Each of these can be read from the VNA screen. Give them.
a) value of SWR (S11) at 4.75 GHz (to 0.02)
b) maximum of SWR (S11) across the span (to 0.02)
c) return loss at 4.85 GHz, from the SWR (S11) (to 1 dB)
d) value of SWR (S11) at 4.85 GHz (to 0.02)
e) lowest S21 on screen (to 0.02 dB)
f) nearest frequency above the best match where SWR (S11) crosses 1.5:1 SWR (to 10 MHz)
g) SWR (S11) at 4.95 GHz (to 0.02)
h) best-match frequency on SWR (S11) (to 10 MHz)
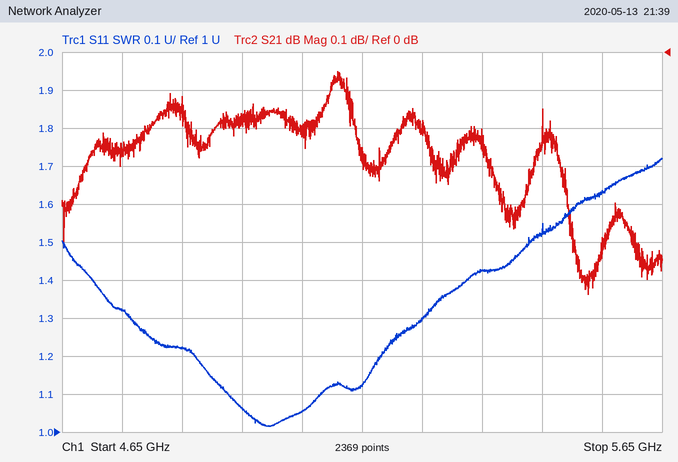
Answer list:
1.32
1.72
20 dB
1.22
-0.64 dB
5.43 GHz
1.06
4.99 GHz
